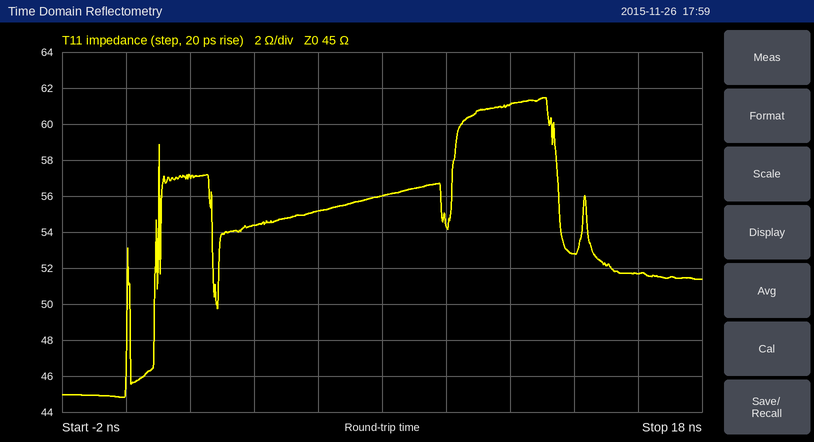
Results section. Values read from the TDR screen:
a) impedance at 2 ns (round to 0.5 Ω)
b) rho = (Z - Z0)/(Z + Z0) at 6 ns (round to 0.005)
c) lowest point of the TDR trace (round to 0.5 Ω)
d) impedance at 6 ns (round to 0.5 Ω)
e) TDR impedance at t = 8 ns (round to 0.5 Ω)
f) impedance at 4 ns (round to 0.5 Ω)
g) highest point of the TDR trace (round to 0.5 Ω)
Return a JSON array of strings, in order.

["57.0 Ω", "+0.100", "45.0 Ω", "55.0 Ω", "56.0 Ω", "54.5 Ω", "61.5 Ω"]
